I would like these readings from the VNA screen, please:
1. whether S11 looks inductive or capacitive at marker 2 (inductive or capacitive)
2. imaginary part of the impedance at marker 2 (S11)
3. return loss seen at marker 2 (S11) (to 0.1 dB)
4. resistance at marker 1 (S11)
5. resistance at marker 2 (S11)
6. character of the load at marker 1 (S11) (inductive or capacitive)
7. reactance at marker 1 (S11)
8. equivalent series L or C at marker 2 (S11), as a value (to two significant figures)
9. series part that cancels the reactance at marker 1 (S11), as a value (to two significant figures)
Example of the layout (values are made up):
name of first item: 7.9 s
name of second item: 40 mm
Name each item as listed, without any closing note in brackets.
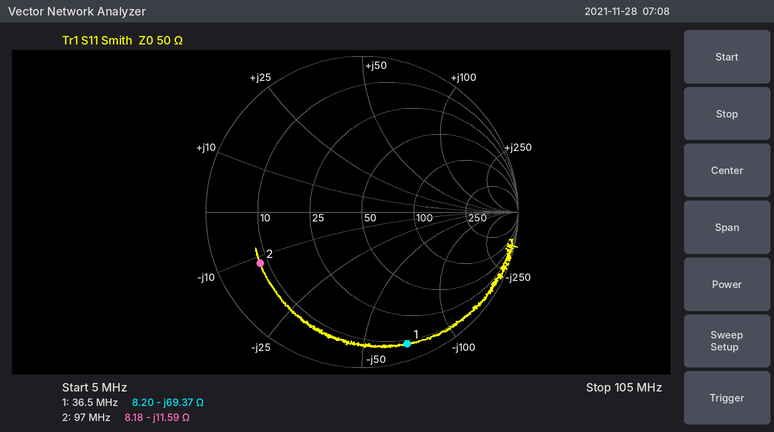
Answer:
whether S11 looks inductive or capacitive at marker 2: capacitive
imaginary part of the impedance at marker 2: -11.59 Ω
return loss seen at marker 2 (S11): 2.7 dB
resistance at marker 1: 8.20 Ω
resistance at marker 2: 8.18 Ω
character of the load at marker 1 (S11): capacitive
reactance at marker 1: -69.37 Ω
equivalent series L or C at marker 2 (S11), as a value: 140 pF
series part that cancels the reactance at marker 1 (S11), as a value: 300 nH
